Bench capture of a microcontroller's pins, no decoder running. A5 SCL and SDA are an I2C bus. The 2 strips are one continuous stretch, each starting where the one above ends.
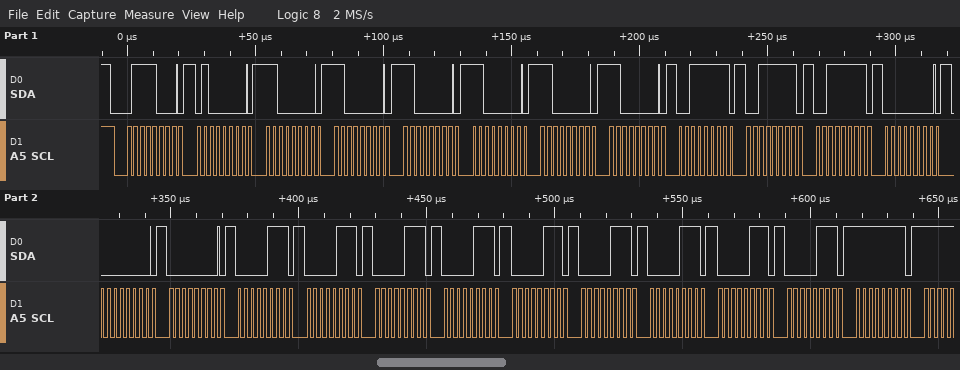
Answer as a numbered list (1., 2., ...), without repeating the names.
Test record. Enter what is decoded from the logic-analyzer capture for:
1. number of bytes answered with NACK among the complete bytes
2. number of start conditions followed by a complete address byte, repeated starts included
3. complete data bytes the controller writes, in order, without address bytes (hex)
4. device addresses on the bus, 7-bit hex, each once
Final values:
1. 0
2. 1
3. 40 C0 C0 C0 C0 C0 C0 3F 3F 3F 00 00 00 07 07 07 07 07 07 07 07 07 FF
4. 0x3C
